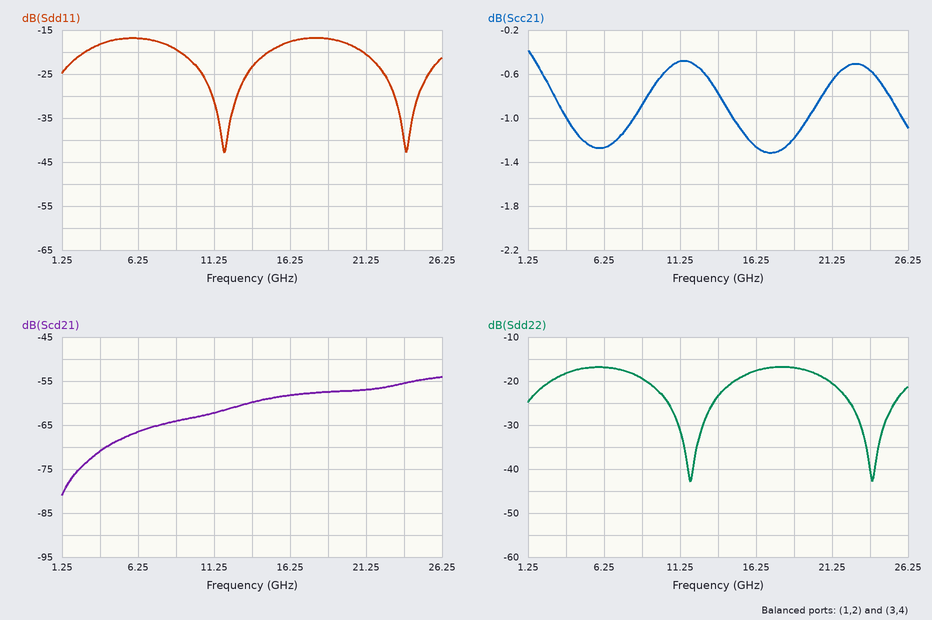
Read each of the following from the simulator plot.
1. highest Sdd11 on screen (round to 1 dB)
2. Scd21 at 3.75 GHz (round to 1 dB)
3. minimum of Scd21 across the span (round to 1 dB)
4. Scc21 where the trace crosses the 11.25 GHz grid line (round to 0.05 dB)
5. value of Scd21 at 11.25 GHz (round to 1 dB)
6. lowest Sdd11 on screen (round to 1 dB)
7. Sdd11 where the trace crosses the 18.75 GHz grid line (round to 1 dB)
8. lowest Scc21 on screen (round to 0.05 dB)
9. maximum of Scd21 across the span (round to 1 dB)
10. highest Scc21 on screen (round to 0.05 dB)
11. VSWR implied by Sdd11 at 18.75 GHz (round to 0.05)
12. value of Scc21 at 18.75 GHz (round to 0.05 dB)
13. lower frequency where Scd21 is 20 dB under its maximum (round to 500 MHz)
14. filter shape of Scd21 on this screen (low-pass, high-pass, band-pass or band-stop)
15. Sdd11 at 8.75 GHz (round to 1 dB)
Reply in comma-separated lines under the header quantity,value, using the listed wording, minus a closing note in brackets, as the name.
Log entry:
quantity,value
highest Sdd11 on screen,-17 dB
Scd21 at 3.75 GHz,-71 dB
minimum of Scd21 across the span,-81 dB
Scc21 where the trace crosses the 11.25 GHz grid line,-0.50 dB
value of Scd21 at 11.25 GHz,-62 dB
lowest Sdd11 on screen,-43 dB
Sdd11 where the trace crosses the 18.75 GHz grid line,-17 dB
lowest Scc21 on screen,-1.30 dB
maximum of Scd21 across the span,-54 dB
highest Scc21 on screen,-0.40 dB
VSWR implied by Sdd11 at 18.75 GHz,1.35
value of Scc21 at 18.75 GHz,-1.20 dB
lower frequency where Scd21 is 20 dB under its maximum,2.5 GHz
filter shape of Scd21 on this screen,high-pass
Sdd11 at 8.75 GHz,-19 dB
